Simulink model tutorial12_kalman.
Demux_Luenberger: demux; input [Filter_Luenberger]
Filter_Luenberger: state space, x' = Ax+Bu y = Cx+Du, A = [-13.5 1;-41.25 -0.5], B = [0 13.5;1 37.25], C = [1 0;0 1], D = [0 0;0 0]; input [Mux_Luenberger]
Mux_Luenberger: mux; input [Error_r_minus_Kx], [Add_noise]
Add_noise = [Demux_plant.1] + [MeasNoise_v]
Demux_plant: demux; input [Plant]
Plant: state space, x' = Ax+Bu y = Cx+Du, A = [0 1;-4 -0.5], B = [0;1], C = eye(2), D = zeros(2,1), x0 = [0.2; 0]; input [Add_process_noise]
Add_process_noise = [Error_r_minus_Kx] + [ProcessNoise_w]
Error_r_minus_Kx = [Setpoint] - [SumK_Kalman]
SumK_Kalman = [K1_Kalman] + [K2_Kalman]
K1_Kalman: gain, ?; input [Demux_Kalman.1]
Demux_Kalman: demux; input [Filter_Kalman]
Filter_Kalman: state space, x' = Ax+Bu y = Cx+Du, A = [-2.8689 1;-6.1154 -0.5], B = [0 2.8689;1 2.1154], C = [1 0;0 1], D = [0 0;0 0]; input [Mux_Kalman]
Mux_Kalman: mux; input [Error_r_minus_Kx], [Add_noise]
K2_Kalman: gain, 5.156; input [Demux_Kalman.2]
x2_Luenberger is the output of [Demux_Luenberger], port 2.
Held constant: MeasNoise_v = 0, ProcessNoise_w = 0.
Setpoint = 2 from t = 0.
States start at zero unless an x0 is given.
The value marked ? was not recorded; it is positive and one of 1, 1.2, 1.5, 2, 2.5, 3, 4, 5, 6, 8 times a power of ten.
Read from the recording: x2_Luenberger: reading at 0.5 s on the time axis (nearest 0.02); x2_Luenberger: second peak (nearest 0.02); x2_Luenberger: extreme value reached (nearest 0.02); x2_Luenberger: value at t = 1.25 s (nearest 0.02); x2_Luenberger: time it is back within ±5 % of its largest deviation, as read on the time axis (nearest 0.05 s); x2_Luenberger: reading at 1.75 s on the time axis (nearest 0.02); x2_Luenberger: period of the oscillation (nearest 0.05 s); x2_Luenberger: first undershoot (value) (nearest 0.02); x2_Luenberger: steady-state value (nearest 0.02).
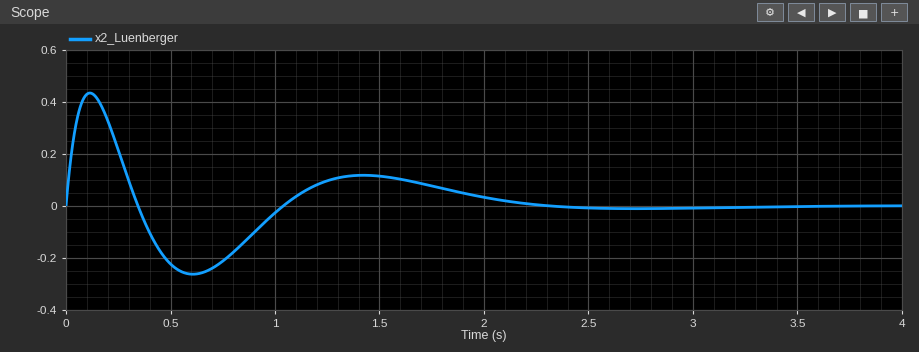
-0.22
0.12
0.44
0.10
2.10 s
0.08
1.30 s
-0.26
0.00
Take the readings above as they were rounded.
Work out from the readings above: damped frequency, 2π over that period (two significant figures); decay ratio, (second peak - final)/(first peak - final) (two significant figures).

4.8 rad/s
0.27
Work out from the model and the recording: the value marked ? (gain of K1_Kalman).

20
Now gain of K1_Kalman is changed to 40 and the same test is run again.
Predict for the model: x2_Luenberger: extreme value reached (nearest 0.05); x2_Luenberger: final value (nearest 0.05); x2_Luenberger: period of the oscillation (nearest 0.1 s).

0.40
0.00
1.0 s
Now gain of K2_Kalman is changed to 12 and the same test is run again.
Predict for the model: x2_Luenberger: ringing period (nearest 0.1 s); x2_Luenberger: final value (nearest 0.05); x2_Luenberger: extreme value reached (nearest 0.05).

1.5 s
0.00
0.40
